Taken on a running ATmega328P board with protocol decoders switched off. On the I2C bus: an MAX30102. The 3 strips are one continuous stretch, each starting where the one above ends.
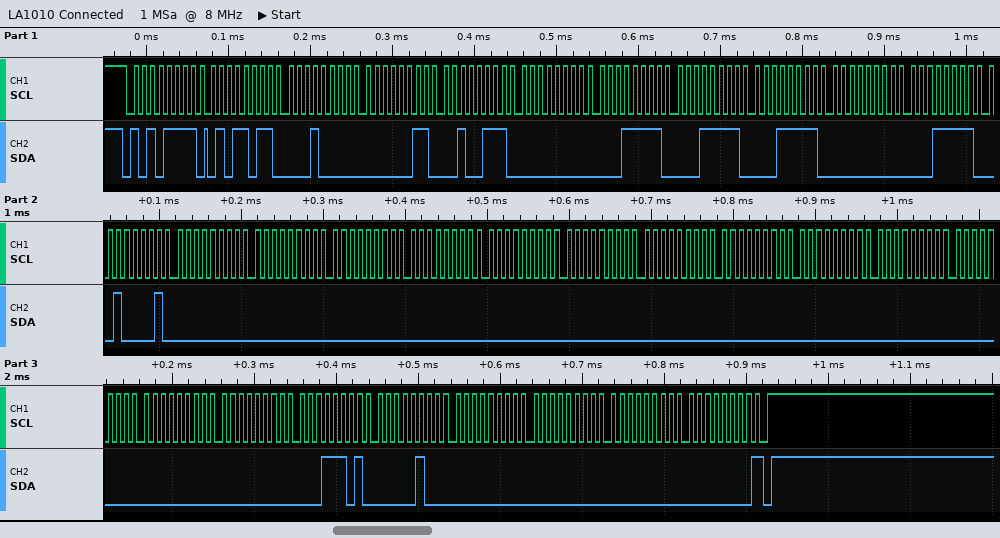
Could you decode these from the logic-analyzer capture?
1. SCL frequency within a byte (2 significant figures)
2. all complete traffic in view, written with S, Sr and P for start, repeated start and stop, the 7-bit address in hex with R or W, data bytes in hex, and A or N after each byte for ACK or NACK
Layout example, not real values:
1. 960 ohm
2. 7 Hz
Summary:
1. 100 kHz
2. S 57R A 5B A 10 A 03 A 27 A 00 A 1F A 1F A 1F A 00 A 1F A 21 A 00 A 00 A 00 A 00 A 00 A 00 A 00 A 00 A 00 A 00 A 00 A 00 A 00 A 1D A 04 A 00 A 00 A 00 A 00 N P
